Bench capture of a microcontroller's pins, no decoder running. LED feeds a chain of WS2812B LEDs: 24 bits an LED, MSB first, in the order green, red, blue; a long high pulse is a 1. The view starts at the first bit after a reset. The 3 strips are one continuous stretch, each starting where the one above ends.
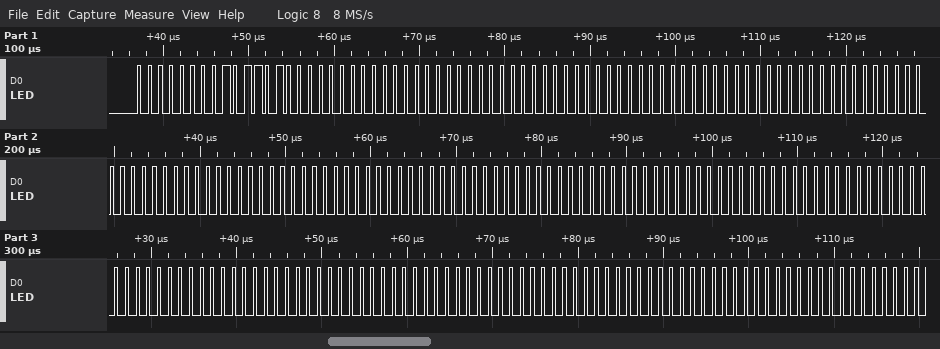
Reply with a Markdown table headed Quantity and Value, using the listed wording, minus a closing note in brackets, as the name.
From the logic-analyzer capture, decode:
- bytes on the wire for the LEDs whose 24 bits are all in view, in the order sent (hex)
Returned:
| Quantity | Value |
|---|---|
| bytes on the wire for the LEDs whose 24 bits are all in view, in the order sent | 00 B4 00 00 00 00 00 00 00 00 00 00 00 00 00 00 00 00 00 00 00 00 00 00 00 00 00 |
